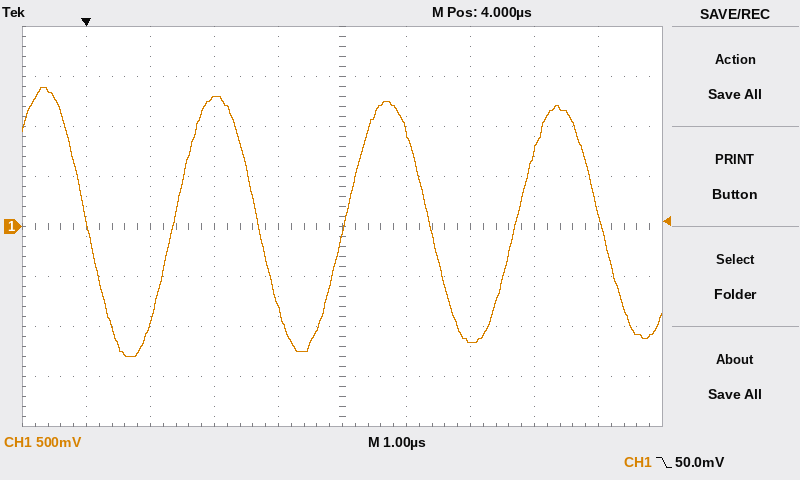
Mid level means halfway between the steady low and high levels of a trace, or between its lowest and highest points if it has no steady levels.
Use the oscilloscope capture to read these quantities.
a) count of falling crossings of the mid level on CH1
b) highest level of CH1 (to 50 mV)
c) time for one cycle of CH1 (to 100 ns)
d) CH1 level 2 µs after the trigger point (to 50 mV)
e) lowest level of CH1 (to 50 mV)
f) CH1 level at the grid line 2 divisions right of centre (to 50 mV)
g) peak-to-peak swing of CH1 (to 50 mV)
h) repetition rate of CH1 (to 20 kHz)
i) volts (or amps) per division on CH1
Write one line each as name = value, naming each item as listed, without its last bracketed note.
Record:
count of falling crossings of the mid level on CH1 = 4
highest level of CH1 = 1.40 V
time for one cycle of CH1 = 2.7 µs
CH1 level 2 µs after the trigger point = 1.30 V
lowest level of CH1 = -1.30 V
CH1 level at the grid line 2 divisions right of centre = -1.15 V
peak-to-peak swing of CH1 = 2.70 V
repetition rate of CH1 = 380 kHz
volts (or amps) per division on CH1 = 500 mV
